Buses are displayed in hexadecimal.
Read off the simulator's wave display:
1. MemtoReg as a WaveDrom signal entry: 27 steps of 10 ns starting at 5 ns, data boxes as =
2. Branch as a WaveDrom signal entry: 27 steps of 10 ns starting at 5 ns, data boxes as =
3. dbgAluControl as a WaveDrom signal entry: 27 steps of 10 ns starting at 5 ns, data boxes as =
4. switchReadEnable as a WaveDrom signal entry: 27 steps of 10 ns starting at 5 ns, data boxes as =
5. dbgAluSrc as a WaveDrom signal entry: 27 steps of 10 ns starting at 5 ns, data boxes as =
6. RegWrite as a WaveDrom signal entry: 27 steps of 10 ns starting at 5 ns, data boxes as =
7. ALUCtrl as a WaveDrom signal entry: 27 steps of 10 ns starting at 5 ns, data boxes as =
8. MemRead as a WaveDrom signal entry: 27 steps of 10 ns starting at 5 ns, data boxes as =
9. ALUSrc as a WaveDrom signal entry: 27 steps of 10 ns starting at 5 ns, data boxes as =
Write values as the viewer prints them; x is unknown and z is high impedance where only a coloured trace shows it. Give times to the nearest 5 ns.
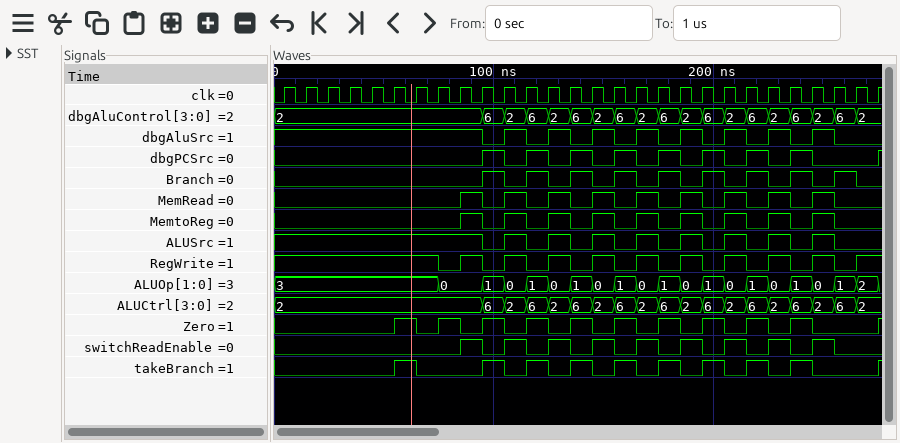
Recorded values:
{name: 'MemtoReg', wave: '0.......101010101010101010.'}
{name: 'Branch', wave: '0........101010101010101010'}
{name: 'dbgAluControl', wave: '=........==================', data: '2 6 2 6 2 6 2 6 2 6 2 6 2 6 2 6 2 6 2'}
{name: 'switchReadEnable', wave: '0.......101010101010101010.'}
{name: 'dbgAluSrc', wave: '1........01010101010101010.'}
{name: 'RegWrite', wave: '1......01010101010101010101'}
{name: 'ALUCtrl', wave: '=........==================', data: '2 6 2 6 2 6 2 6 2 6 2 6 2 6 2 6 2 6 2'}
{name: 'MemRead', wave: '0.......101010101010101010.'}
{name: 'ALUSrc', wave: '1........01010101010101010.'}
